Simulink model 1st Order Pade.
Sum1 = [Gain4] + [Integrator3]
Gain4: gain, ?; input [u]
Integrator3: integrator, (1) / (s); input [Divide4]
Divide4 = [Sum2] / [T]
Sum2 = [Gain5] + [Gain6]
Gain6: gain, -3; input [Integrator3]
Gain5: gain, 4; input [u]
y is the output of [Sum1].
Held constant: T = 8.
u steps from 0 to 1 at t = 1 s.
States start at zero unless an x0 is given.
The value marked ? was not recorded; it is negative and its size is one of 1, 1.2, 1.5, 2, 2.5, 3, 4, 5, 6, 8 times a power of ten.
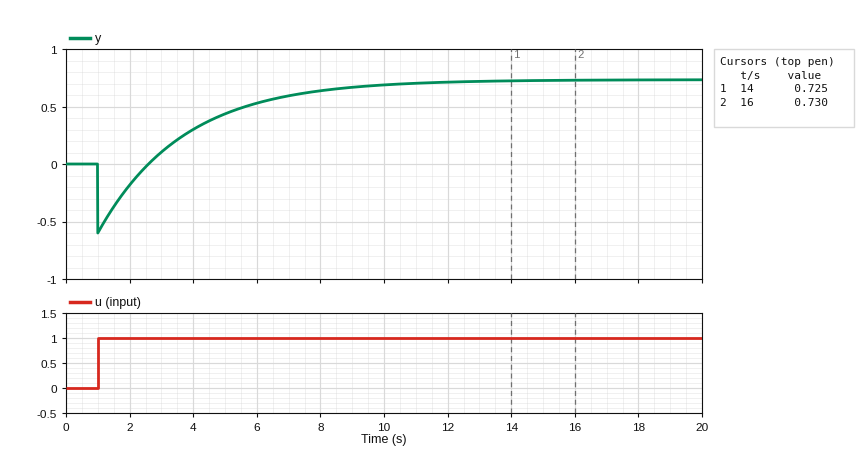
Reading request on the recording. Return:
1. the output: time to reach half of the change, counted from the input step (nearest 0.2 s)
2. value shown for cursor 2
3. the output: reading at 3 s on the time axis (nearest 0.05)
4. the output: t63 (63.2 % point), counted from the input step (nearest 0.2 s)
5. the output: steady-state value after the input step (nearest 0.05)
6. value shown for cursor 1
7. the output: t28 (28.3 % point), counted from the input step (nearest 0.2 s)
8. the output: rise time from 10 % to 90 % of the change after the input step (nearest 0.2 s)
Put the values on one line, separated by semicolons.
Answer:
3.4 s; 0.730; 0.10; 4.2 s; 0.75; 0.725; 2.4 s; 5.8 s
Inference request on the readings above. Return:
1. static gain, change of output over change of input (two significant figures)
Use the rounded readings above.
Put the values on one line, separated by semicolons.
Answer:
0.75
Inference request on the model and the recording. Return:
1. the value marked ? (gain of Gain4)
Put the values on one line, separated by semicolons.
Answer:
-0.6
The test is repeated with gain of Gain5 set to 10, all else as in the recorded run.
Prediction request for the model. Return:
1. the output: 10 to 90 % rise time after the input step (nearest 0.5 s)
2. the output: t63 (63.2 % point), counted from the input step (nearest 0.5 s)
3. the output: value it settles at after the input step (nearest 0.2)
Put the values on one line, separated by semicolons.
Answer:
6.0 s; 3.0 s; 2.8
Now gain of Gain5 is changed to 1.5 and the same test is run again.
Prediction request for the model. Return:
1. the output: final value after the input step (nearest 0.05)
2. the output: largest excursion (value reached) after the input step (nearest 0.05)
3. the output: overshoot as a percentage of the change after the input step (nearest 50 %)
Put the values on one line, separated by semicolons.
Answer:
-0.10; -0.60; 500 %
